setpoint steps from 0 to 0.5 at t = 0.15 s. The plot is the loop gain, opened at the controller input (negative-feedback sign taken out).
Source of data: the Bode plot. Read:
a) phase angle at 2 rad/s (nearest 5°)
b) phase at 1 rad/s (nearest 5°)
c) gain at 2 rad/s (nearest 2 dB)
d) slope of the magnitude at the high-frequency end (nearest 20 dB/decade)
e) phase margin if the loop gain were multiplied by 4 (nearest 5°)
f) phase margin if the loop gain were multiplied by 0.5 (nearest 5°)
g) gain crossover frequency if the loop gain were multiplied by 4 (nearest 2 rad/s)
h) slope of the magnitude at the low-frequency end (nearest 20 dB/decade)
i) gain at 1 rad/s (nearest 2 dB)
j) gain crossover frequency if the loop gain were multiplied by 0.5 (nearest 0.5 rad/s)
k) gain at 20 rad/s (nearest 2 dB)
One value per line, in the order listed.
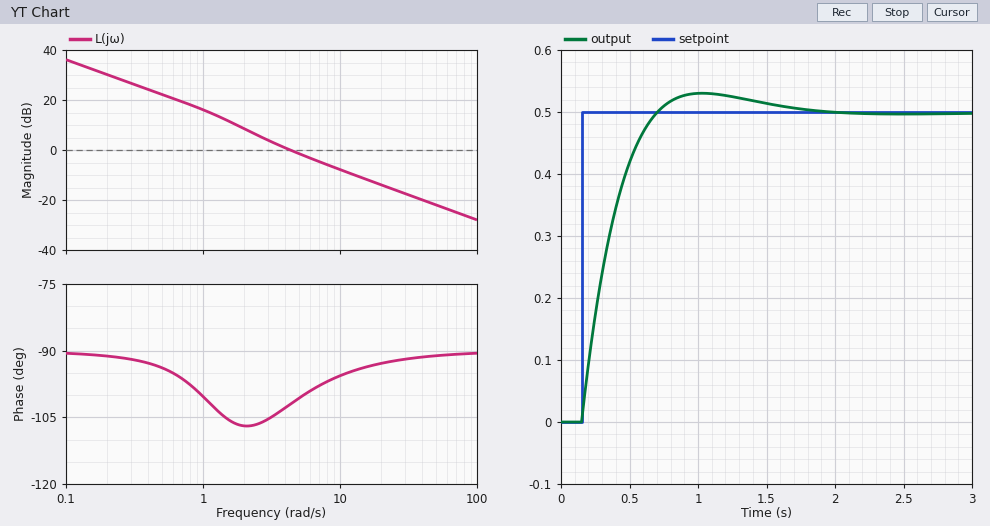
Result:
-105°
-100°
8 dB
-20 dB/decade
85°
75°
16 rad/s
-20 dB/decade
16 dB
2.5 rad/s
-14 dB
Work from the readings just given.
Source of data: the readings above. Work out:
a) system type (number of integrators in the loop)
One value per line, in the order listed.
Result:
1
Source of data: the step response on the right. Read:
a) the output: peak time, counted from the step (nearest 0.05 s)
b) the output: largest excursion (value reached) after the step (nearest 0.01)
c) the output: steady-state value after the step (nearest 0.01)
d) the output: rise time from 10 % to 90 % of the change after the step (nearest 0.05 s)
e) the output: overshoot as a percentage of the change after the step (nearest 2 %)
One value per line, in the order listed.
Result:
0.90 s
0.53
0.50
0.40 s
6 %
